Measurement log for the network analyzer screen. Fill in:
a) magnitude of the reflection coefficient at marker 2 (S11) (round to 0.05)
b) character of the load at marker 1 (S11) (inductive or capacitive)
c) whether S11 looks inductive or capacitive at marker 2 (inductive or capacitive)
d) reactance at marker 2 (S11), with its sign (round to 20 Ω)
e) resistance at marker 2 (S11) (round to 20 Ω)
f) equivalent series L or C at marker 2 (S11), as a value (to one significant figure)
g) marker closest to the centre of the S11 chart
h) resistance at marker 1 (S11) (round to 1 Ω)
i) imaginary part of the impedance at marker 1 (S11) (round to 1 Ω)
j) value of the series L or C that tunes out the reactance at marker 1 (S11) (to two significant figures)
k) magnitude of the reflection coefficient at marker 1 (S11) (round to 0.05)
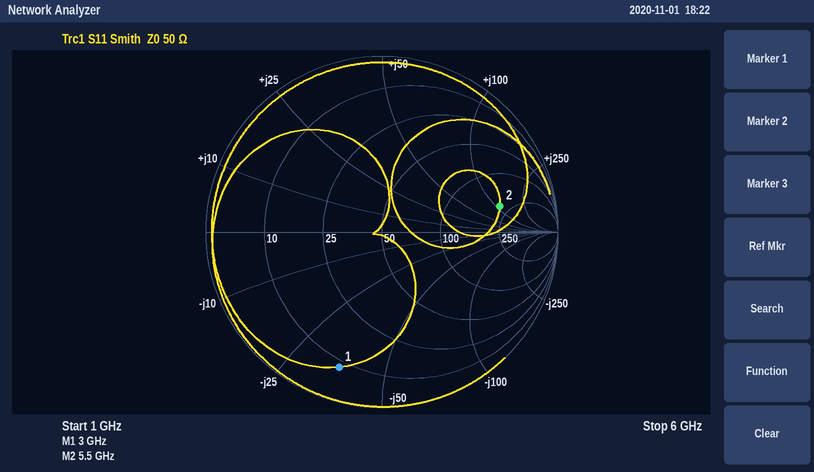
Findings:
0.70
capacitive
inductive
+120 Ω
200 Ω
3 nH
marker 2
8 Ω
-36 Ω
1.9 nH
0.80
